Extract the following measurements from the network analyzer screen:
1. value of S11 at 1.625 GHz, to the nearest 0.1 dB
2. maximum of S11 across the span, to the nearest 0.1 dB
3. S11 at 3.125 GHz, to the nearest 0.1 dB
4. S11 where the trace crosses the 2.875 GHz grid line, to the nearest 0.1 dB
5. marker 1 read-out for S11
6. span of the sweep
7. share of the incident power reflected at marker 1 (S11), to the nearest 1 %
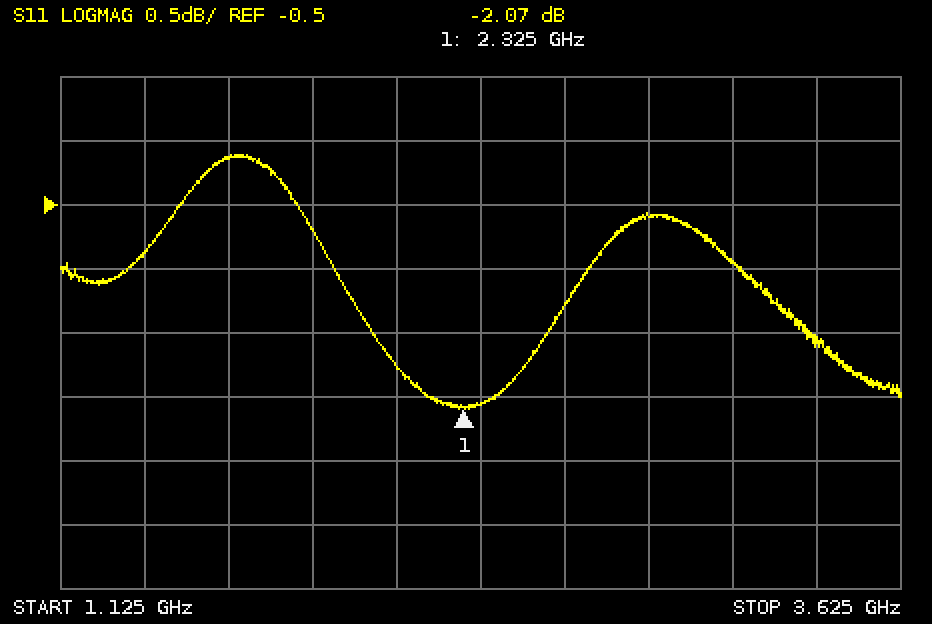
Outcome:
-0.1 dB
-0.1 dB
-0.9 dB
-0.6 dB
-2.07 dB
2.5 GHz
62 %
